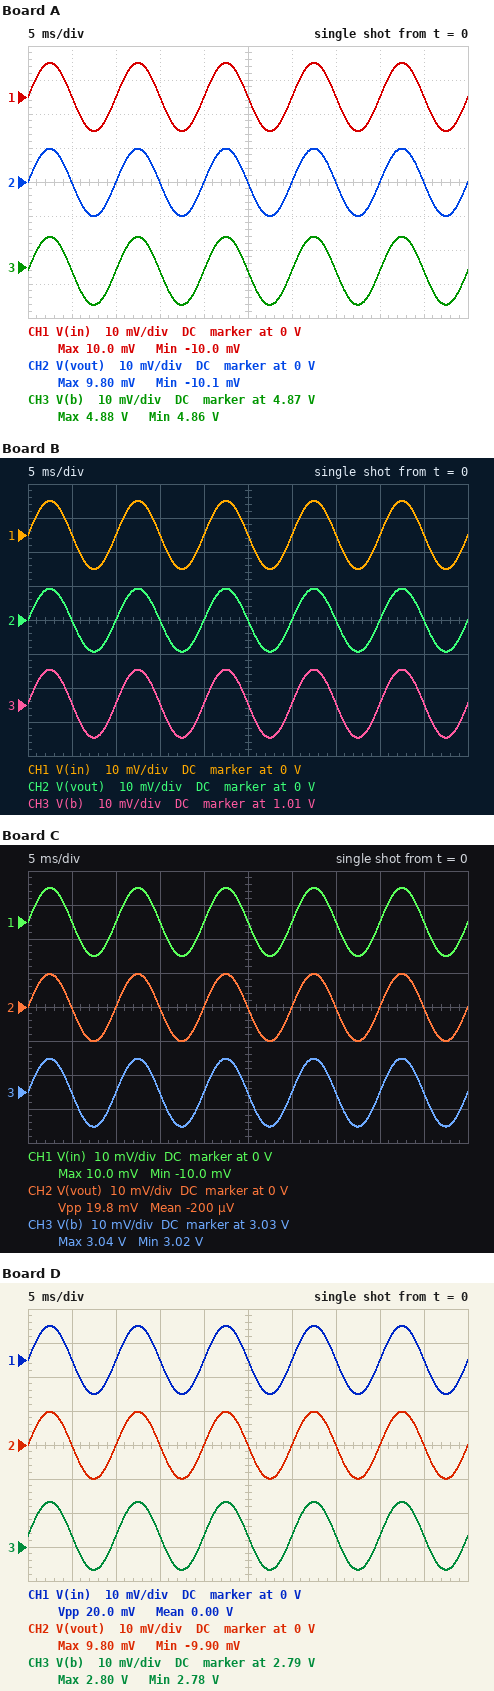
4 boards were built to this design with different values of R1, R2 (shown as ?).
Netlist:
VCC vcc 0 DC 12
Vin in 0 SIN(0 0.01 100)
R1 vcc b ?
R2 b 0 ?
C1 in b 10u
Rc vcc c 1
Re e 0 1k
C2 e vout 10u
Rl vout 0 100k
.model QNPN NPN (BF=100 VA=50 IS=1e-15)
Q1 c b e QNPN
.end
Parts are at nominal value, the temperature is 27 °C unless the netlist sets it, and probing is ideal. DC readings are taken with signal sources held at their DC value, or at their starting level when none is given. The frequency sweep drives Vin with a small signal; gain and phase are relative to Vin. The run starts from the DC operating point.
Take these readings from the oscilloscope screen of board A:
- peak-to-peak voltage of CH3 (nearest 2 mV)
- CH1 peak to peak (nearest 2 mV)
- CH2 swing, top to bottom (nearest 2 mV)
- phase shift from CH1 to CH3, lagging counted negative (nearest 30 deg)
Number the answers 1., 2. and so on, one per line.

1. 20 mV
2. 20 mV
3. 20 mV
4. 0 deg
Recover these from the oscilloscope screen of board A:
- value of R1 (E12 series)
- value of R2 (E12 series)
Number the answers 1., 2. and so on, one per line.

1. 33 kΩ
2. 27 kΩ
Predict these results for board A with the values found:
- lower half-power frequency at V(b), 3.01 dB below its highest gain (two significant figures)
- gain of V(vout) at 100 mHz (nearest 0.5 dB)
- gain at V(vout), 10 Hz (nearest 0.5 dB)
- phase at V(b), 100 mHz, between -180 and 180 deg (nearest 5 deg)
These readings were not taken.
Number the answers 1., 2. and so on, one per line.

1. 1.2 Hz
2. -27.5 dB
3. 0 dB
4. 85 deg
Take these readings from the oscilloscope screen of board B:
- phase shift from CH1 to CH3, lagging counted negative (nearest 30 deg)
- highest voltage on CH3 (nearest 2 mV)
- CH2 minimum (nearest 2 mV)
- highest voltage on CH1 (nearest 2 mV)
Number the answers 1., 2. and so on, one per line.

1. 0 deg
2. 1.020 V
3. -10 mV
4. 10 mV
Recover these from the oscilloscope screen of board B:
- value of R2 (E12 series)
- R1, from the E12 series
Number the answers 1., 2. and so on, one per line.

1. 33 kΩ
2. 330 kΩ
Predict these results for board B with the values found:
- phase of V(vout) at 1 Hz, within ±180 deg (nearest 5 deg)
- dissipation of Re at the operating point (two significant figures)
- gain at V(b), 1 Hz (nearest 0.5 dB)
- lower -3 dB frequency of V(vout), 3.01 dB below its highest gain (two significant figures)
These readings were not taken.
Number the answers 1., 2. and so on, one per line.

1. 40 deg
2. 110 µW
3. -1.5 dB
4. 690 mHz
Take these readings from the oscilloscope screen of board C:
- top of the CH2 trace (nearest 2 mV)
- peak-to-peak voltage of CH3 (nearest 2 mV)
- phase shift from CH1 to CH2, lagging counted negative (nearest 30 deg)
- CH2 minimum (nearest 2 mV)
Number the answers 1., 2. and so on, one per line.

1. 10 mV
2. 20 mV
3. 0 deg
4. -10 mV
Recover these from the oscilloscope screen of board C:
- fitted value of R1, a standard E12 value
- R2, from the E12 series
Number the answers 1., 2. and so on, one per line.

1. 33 kΩ
2. 12 kΩ
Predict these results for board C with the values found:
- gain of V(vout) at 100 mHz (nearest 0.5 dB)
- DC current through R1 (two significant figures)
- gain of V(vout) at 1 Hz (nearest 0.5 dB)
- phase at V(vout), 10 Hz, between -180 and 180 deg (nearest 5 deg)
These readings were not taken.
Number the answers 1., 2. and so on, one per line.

1. -31.5 dB
2. 270 µA
3. -7.0 dB
4. 10 deg
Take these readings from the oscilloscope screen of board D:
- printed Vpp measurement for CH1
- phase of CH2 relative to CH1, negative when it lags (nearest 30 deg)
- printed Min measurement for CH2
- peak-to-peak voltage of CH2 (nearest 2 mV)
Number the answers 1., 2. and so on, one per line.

1. 20.0 mV
2. 0 deg
3. -9.90 mV
4. 20 mV
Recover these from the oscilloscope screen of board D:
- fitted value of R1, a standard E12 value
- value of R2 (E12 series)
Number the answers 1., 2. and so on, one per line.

1. 120 kΩ
2. 47 kΩ
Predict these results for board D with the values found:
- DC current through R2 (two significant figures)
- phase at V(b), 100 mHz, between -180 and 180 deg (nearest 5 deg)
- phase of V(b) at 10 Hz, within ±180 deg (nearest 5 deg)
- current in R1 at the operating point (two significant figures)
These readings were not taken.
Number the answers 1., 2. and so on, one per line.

1. 59 µA
2. 80 deg
3. 5 deg
4. 77 µA
